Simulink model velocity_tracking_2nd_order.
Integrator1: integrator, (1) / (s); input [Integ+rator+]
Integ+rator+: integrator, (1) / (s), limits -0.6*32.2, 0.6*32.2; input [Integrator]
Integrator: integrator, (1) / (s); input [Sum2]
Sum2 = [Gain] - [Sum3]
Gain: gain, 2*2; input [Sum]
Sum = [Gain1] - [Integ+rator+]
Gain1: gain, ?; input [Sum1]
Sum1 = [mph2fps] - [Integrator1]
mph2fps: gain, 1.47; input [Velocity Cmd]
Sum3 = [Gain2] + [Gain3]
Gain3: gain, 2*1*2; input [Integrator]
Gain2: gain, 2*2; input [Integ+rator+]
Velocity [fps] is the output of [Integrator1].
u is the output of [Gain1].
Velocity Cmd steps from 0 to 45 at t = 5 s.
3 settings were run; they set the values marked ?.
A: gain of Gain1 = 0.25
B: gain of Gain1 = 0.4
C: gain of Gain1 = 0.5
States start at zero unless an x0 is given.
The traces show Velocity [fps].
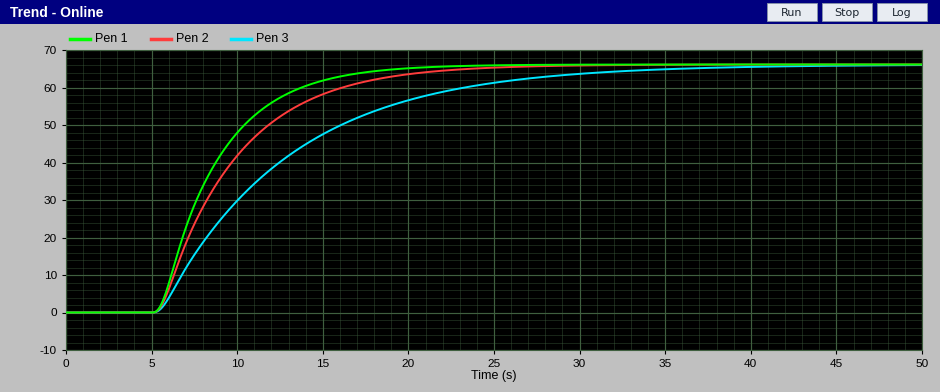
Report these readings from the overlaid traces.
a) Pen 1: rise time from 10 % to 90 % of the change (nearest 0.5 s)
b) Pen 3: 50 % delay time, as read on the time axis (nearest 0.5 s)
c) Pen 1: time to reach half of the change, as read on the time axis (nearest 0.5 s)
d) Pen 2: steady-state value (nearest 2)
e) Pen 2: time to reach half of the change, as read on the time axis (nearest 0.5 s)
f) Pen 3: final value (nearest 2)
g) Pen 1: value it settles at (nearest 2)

7.5 s
10.5 s
8.0 s
66
8.5 s
66
66
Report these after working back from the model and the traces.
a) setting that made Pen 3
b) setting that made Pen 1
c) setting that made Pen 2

A
C
B
